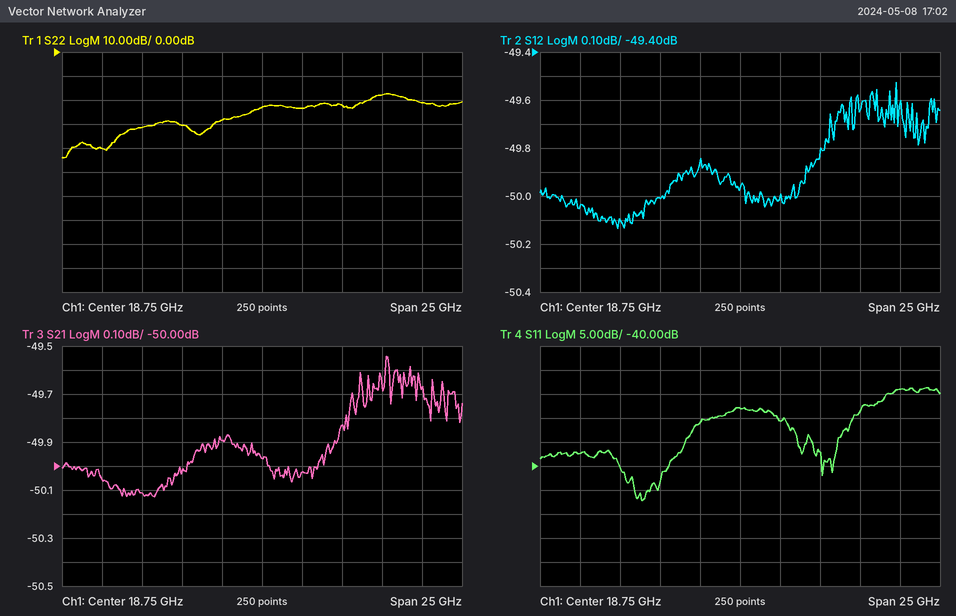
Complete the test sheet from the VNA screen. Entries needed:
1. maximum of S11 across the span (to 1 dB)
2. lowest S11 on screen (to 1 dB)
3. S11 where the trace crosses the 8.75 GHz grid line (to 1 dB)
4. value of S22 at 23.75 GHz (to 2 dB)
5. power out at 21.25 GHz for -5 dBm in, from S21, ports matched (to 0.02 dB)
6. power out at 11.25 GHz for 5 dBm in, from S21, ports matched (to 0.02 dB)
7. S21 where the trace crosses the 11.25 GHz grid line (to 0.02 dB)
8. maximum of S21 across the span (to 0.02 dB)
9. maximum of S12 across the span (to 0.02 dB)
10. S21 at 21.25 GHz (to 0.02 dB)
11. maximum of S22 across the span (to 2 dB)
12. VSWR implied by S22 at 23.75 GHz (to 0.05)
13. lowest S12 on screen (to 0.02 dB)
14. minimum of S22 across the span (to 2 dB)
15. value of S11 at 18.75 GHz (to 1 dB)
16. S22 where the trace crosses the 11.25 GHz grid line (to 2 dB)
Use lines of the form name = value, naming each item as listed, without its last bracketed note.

maximum of S11 across the span = -24 dB
lowest S11 on screen = -47 dB
S11 where the trace crosses the 8.75 GHz grid line = -37 dB
value of S22 at 23.75 GHz = -22 dB
power out at 21.25 GHz for -5 dBm in, from S21, ports matched = -55.02 dBm
power out at 11.25 GHz for 5 dBm in, from S21, ports matched = -45.12 dBm
S21 where the trace crosses the 11.25 GHz grid line = -50.12 dB
maximum of S21 across the span = -49.54 dB
maximum of S12 across the span = -49.52 dB
S21 at 21.25 GHz = -50.02 dB
maximum of S22 across the span = -18 dB
VSWR implied by S22 at 23.75 GHz = 1.15
lowest S12 on screen = -50.14 dB
minimum of S22 across the span = -44 dB
value of S11 at 18.75 GHz = -28 dB
S22 where the trace crosses the 11.25 GHz grid line = -32 dB
